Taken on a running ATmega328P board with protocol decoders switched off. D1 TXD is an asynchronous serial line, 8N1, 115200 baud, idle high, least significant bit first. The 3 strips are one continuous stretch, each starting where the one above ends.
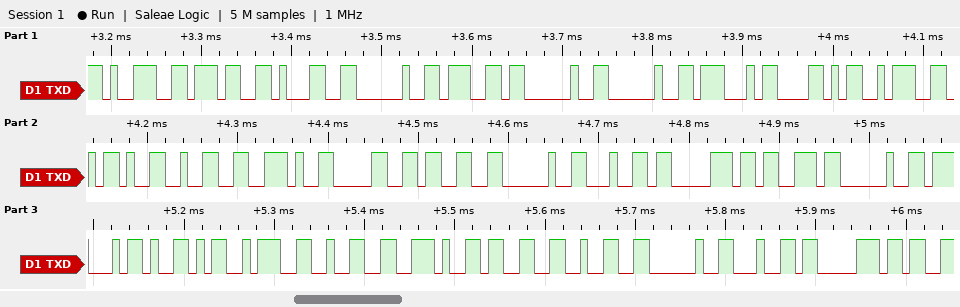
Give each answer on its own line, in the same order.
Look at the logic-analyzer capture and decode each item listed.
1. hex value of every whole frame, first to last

39 37 31 20 67 20 20 47 58 3A 2D 32 2E 30 33 20 64 70 73 20 47 59 3A 32 2E 33 32 20 64 70
